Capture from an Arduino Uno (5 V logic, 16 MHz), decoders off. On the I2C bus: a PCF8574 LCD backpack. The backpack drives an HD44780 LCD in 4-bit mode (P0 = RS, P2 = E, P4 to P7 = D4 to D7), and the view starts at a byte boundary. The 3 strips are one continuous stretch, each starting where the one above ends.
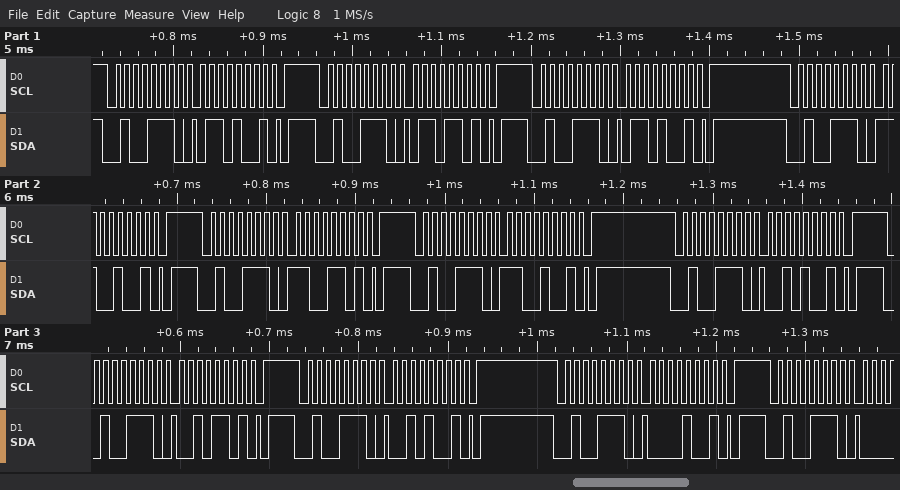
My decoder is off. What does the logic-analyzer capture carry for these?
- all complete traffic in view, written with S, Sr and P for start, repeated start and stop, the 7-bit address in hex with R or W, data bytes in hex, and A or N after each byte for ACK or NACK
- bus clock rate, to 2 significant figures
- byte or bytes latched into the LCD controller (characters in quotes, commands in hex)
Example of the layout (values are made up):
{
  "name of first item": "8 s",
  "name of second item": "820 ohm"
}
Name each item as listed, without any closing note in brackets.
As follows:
{
  "all complete traffic in view, written with S, Sr and P for start, repeated start and stop, the 7-bit address in hex with R or W, data bytes in hex, and A or N after each byte for ACK or NACK": "S 27W A 69 A P S 27W A 6D A P S 27W A 69 A P S 27W A C9 A P S 27W A CD A P S 27W A C9 A P S 27W A 29 A P S 27W A 2D A P S 27W A 29 A P S 27W A 09 A P S 27W A",
  "bus clock rate, to 2 significant figures": "100 kHz",
  "byte or bytes latched into the LCD controller": "'l'"
}
